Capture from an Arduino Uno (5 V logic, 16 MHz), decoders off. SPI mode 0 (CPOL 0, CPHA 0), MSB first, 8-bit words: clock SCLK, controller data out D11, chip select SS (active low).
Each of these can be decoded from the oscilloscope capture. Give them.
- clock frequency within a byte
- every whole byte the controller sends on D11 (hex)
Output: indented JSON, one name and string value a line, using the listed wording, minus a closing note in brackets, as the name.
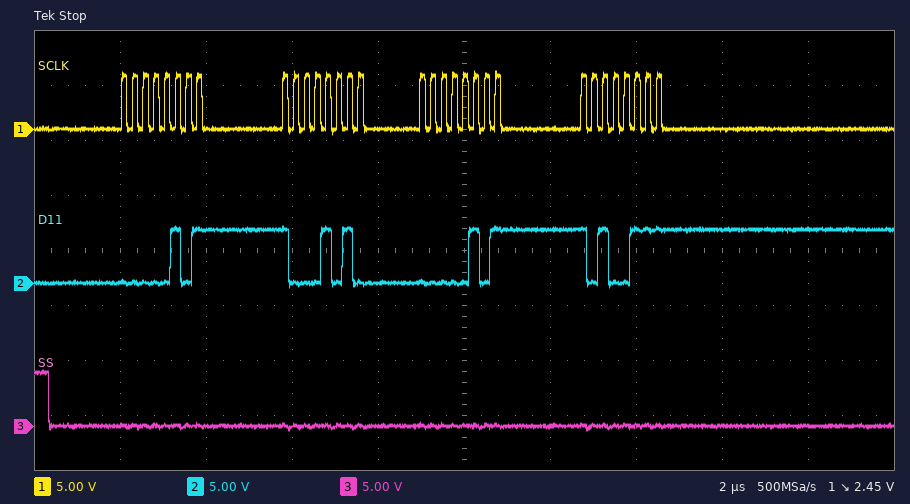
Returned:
{
  "clock frequency within a byte": "4 MHz",
  "every whole byte the controller sends on D11": "0x05 0x8A 0x05 0xA7"
}
